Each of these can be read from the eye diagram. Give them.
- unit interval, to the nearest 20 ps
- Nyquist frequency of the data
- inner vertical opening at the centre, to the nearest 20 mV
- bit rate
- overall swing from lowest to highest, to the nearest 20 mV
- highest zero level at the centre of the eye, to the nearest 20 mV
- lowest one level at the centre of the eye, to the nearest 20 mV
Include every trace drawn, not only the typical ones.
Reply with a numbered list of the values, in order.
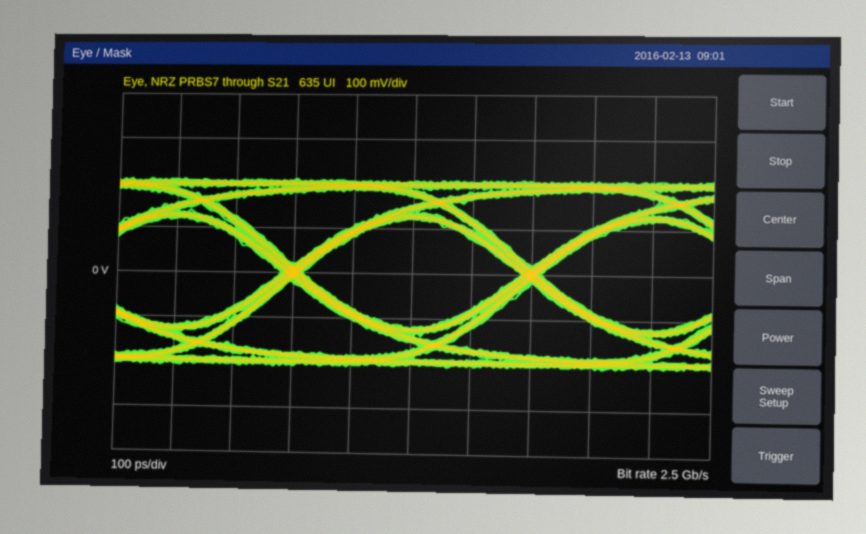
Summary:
1. 400 ps
2. 1.25 GHz
3. 240 mV
4. 2.5 Gb/s
5. 420 mV
6. -120 mV
7. 120 mV
